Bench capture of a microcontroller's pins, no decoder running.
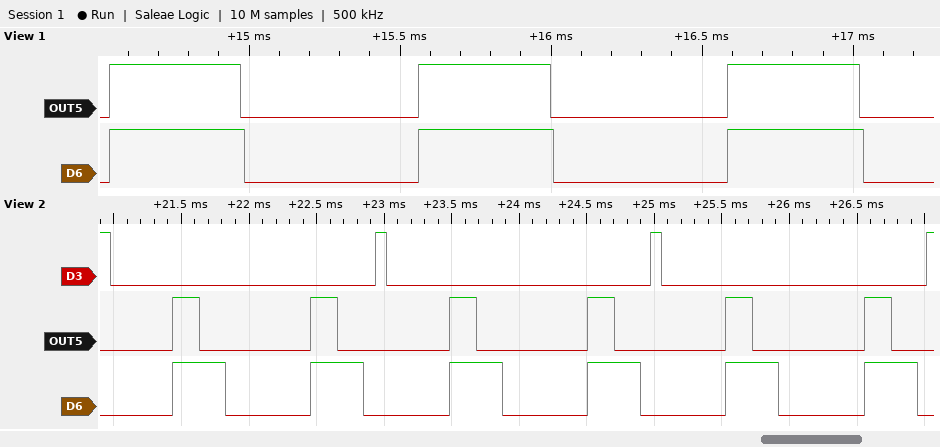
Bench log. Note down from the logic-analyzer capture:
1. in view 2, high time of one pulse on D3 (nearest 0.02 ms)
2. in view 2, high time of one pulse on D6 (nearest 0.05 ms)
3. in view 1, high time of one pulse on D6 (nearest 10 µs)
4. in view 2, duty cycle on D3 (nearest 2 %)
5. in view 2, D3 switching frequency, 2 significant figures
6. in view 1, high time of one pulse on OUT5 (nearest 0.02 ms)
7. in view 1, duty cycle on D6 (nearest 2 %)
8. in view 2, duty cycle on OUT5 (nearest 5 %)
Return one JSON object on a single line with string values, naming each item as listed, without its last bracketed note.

{"in view 2, high time of one pulse on D3": "0.08 ms", "in view 2, high time of one pulse on D6": "0.40 ms", "in view 1, high time of one pulse on D6": "450 µs", "in view 2, duty cycle on D3": "4 %", "in view 2, D3 switching frequency, 2 significant figures": "490 Hz", "in view 1, high time of one pulse on OUT5": "0.44 ms", "in view 1, duty cycle on D6": "44 %", "in view 2, duty cycle on OUT5": "20 %"}
